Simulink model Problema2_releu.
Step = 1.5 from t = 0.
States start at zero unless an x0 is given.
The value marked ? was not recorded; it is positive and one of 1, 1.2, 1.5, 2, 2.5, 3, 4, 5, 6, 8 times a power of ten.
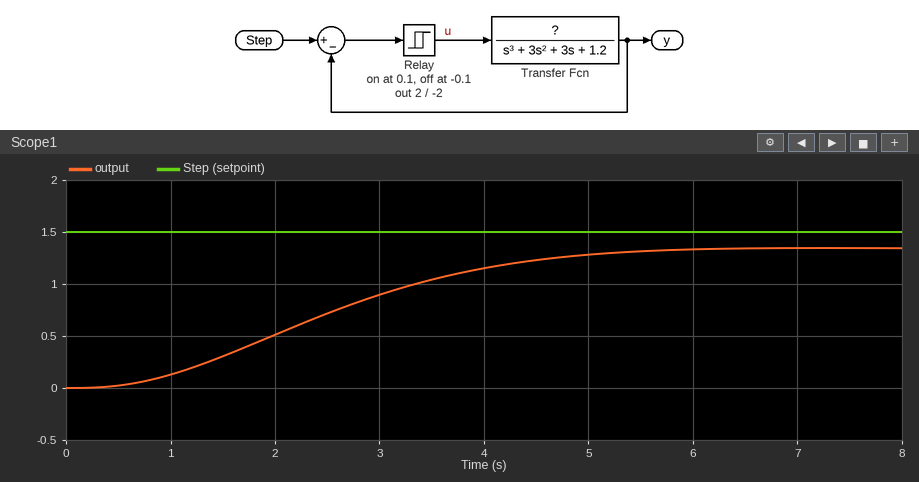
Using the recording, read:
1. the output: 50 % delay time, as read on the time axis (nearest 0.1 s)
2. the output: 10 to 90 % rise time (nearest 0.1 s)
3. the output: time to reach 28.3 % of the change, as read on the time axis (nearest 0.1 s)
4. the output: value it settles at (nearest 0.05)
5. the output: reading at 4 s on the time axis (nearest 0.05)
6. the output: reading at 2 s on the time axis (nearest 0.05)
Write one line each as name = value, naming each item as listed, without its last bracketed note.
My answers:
the output: 50 % delay time, as read on the time axis = 2.4 s
the output: 10 to 90 % rise time = 3.3 s
the output: time to reach 28.3 % of the change, as read on the time axis = 1.7 s
the output: value it settles at = 1.35
the output: reading at 4 s on the time axis = 1.15
the output: reading at 2 s on the time axis = 0.50
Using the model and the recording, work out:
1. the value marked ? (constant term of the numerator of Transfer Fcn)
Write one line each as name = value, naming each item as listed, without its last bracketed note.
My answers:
the value marked ? = 0.8
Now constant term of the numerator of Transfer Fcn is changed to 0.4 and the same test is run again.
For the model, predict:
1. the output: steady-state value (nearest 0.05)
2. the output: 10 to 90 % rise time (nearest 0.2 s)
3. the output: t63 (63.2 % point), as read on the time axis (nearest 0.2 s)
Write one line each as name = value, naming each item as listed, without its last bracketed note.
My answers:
the output: steady-state value = 0.65
the output: 10 to 90 % rise time = 3.2 s
the output: t63 (63.2 % point), as read on the time axis = 2.8 s
